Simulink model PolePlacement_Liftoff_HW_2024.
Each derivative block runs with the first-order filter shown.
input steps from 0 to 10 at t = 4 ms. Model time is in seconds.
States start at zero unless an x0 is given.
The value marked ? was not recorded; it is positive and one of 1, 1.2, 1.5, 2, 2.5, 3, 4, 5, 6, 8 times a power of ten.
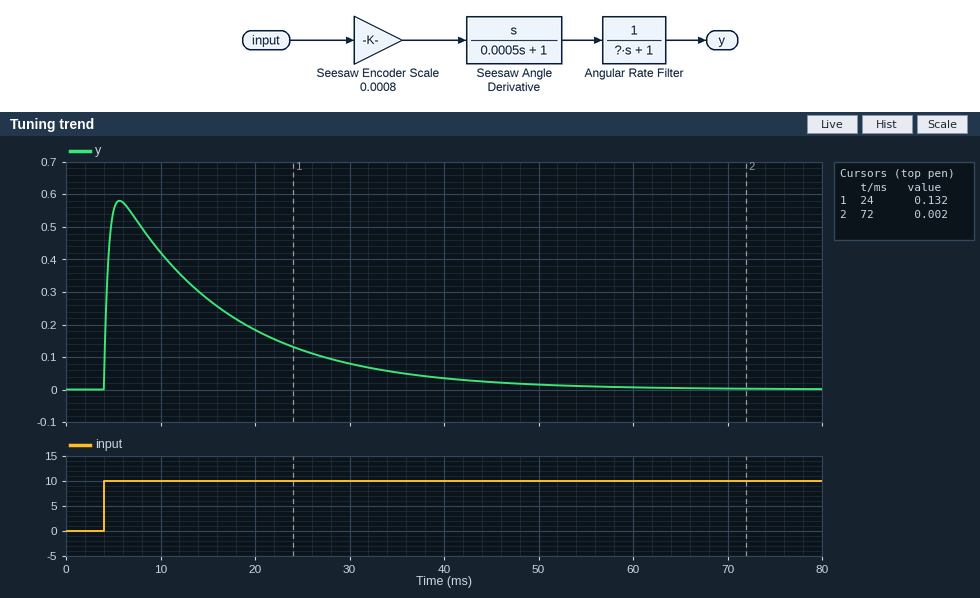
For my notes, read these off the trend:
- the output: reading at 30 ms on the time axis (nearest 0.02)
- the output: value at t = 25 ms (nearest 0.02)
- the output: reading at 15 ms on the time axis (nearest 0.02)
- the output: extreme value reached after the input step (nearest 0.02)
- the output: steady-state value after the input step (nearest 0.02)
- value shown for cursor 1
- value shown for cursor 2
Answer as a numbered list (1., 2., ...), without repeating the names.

1. 0.08
2. 0.12
3. 0.28
4. 0.58
5. 0.00
6. 0.132
7. 0.002
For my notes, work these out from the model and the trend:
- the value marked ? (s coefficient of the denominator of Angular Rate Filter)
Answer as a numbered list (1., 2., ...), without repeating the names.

1. 0.012
